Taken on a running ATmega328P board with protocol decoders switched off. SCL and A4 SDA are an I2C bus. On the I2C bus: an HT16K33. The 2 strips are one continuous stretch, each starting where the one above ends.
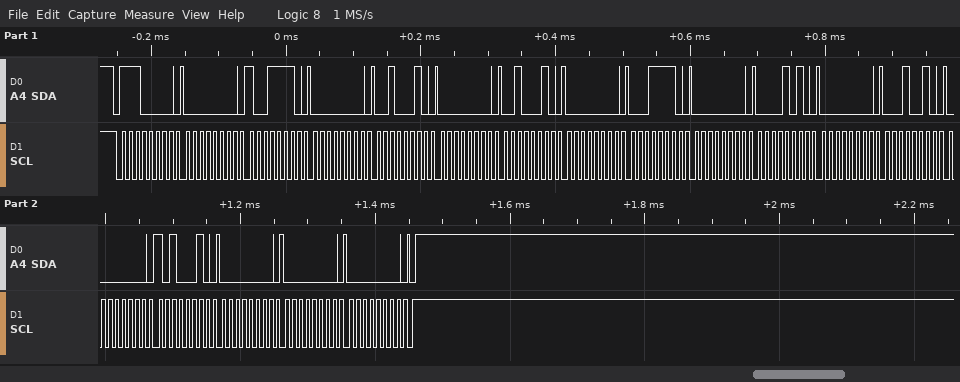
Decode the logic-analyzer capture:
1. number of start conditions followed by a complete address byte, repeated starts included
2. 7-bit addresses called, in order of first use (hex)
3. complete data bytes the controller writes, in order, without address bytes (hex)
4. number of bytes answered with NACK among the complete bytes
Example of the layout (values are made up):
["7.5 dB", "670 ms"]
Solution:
["1", "0x70", "00 9E 00 22 00 22 00 1E 00 0A 00 12 00 A2 00 00 00", "0"]
